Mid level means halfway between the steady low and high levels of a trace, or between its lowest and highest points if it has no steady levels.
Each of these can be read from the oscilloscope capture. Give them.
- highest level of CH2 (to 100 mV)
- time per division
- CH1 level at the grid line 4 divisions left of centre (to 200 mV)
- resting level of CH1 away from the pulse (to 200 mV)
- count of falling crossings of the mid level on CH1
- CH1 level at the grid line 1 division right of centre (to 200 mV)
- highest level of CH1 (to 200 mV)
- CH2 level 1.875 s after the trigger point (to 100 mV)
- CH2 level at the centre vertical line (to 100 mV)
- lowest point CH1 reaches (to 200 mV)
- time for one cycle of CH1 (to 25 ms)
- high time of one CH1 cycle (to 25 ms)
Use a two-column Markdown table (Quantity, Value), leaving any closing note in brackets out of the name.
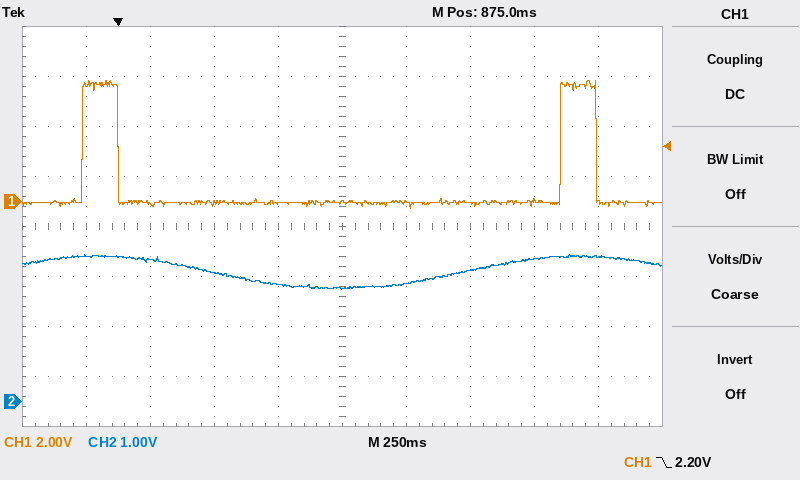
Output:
| Quantity | Value |
|---|---|
| highest level of CH2 | 2.9 V |
| time per division | 250 ms |
| CH1 level at the grid line 4 divisions left of centre | 4.8 V |
| resting level of CH1 away from the pulse | 0.0 V |
| count of falling crossings of the mid level on CH1 | 2 |
| CH1 level at the grid line 1 division right of centre | 0.0 V |
| highest level of CH1 | 4.8 V |
| CH2 level 1.875 s after the trigger point | 2.9 V |
| CH2 level at the centre vertical line | 2.3 V |
| lowest point CH1 reaches | -200 mV |
| time for one cycle of CH1 | 1.875 s |
| high time of one CH1 cycle | 150 ms |
